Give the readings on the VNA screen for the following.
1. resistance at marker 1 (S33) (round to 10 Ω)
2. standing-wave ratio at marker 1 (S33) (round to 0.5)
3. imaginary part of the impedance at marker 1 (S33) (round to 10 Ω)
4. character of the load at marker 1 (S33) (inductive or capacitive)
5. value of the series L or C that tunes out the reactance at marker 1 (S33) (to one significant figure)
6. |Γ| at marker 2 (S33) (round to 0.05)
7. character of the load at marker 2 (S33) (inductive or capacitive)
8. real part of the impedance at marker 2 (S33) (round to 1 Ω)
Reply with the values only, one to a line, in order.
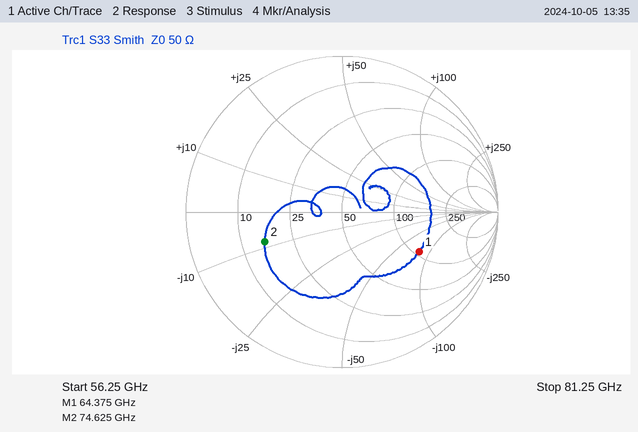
110 Ω
3.5
-80 Ω
capacitive
200 pH
0.55
capacitive
16 Ω
